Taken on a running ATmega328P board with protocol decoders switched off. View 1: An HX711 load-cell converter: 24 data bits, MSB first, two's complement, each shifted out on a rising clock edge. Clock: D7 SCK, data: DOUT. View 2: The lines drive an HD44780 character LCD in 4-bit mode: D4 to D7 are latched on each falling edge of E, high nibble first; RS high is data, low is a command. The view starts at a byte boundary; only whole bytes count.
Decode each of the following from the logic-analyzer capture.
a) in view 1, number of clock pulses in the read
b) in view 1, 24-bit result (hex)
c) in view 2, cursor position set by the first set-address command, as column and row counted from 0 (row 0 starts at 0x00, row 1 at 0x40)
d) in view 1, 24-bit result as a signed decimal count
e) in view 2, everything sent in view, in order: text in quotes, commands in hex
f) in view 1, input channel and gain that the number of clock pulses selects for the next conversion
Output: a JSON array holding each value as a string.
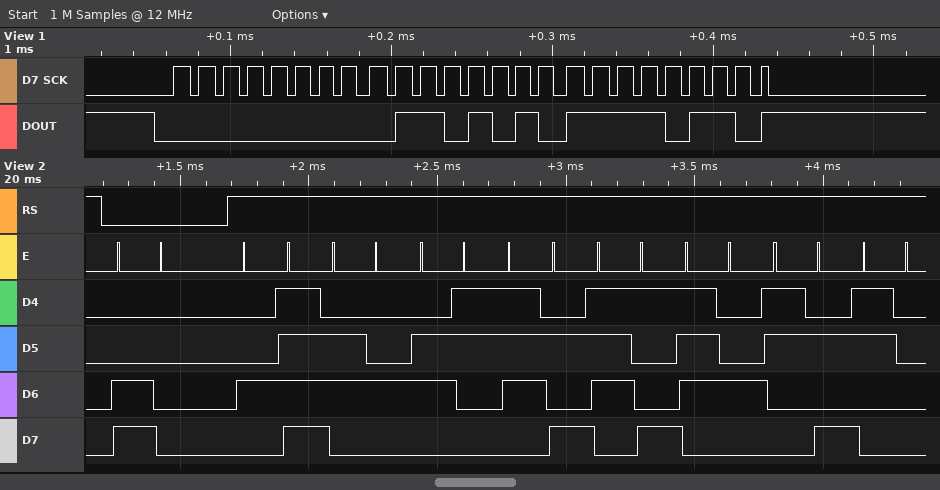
["25", "0x006AF6", "column 0, row 1", "27382", "0xC0 \"Odczyt:0\"", "channel A, gain 128"]
